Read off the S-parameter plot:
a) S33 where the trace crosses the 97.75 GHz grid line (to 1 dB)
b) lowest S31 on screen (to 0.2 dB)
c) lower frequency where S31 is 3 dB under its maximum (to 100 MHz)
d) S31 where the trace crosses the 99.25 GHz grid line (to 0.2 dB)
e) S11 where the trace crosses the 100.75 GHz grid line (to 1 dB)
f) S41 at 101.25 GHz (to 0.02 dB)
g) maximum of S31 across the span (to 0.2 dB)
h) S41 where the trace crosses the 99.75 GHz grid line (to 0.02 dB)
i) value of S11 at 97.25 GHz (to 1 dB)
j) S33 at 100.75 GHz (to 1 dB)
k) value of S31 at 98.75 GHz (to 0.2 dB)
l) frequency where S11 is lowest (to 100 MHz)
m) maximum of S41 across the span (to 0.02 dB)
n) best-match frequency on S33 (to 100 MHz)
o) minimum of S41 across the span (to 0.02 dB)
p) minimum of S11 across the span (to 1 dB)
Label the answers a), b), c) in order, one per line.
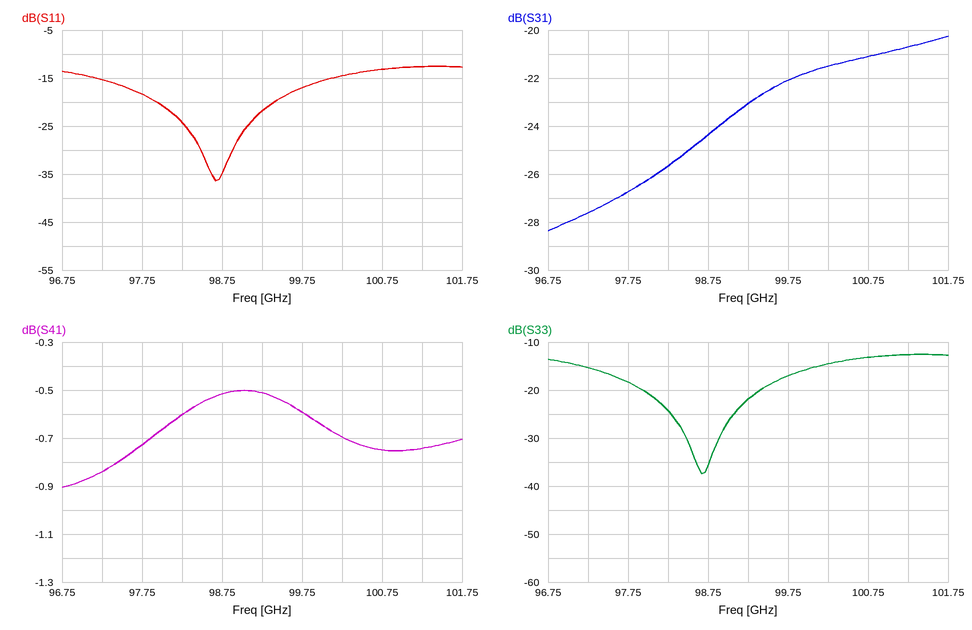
a) -18 dB
b) -28.4 dB
c) 99.2 GHz
d) -23.0 dB
e) -13 dB
f) -0.74 dB
g) -20.2 dB
h) -0.60 dB
i) -15 dB
j) -13 dB
k) -24.4 dB
l) 98.7 GHz
m) -0.50 dB
n) 98.7 GHz
o) -0.90 dB
p) -36 dB
